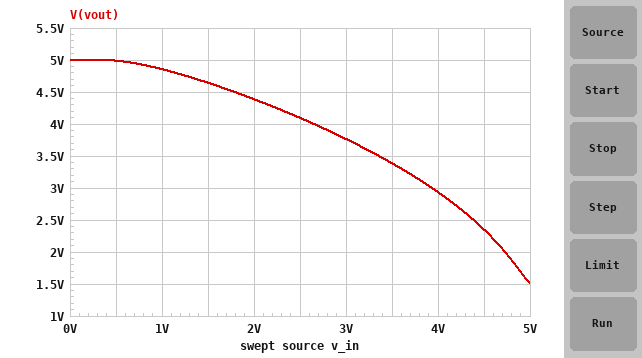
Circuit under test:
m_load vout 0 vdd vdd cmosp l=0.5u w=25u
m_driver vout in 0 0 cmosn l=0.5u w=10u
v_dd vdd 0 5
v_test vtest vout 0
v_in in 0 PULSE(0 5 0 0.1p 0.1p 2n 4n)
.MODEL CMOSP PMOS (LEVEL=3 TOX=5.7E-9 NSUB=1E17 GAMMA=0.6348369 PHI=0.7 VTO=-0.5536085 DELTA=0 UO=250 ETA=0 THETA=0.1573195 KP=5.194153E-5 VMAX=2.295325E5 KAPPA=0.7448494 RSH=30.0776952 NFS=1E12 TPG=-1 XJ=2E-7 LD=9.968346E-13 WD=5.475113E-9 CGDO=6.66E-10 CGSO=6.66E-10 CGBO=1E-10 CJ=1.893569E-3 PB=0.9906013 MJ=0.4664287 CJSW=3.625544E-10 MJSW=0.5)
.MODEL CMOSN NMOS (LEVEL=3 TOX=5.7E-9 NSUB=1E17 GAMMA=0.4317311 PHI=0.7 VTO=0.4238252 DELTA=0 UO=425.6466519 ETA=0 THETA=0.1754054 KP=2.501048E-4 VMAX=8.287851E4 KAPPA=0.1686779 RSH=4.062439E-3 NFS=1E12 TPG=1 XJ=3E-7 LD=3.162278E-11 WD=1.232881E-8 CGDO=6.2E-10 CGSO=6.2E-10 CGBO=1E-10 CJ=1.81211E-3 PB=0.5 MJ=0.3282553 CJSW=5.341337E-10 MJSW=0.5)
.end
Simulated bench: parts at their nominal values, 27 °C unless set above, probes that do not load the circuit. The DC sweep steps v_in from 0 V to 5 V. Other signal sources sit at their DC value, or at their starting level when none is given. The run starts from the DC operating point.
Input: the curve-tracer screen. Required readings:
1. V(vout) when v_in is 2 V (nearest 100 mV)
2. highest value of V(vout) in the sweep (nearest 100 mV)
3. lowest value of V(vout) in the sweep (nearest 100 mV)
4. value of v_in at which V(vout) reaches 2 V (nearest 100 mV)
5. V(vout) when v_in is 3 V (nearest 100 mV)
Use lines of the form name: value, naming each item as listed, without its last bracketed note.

V(vout) when v_in is 2 V: 4.4 V
highest value of V(vout) in the sweep: 5.0 V
lowest value of V(vout) in the sweep: 1.5 V
value of v_in at which V(vout) reaches 2 V: 4.7 V
V(vout) when v_in is 3 V: 3.8 V
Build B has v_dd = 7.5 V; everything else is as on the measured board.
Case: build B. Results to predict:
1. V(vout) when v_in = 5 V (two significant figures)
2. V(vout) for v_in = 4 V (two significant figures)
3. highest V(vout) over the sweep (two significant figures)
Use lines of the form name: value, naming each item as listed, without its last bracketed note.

V(vout) when v_in = 5 V: 5.3 V
V(vout) for v_in = 4 V: 5.9 V
highest V(vout) over the sweep: 7.5 V
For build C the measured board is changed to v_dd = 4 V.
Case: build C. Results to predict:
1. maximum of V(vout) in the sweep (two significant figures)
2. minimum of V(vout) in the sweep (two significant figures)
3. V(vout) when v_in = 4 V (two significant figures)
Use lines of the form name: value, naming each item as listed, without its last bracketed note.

maximum of V(vout) in the sweep: 4.0 V
minimum of V(vout) in the sweep: 730 mV
V(vout) when v_in = 4 V: 1.1 V
